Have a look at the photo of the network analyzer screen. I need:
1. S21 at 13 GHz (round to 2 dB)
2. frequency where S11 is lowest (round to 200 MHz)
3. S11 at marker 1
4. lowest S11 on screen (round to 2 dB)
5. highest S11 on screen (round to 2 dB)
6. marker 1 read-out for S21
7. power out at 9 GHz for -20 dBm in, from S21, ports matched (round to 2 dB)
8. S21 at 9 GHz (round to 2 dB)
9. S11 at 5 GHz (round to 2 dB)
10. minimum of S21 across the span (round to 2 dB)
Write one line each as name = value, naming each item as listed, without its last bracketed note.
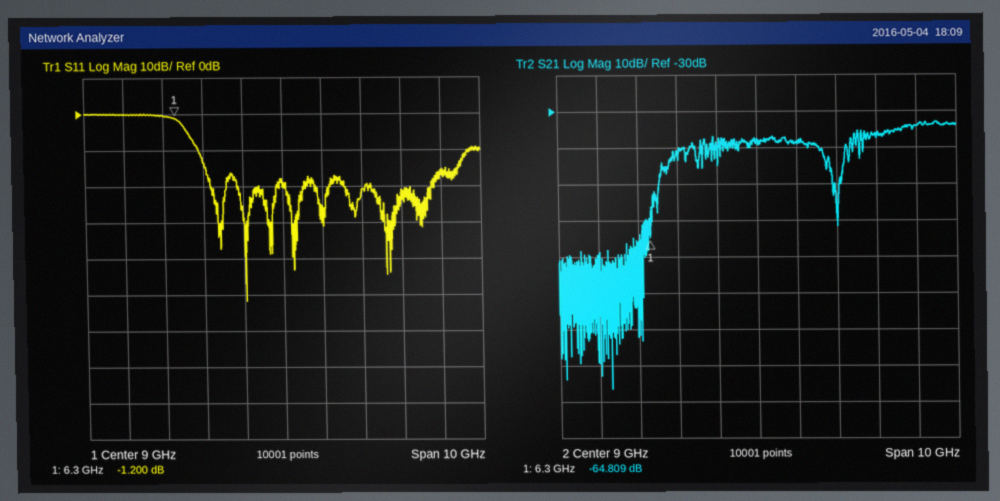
S21 at 13 GHz = -34 dB
frequency where S11 is lowest = 8.0 GHz
S11 at marker 1 = -1.200 dB
lowest S11 on screen = -52 dB
highest S11 on screen = 0 dB
marker 1 read-out for S21 = -64.809 dB
power out at 9 GHz for -20 dBm in, from S21, ports matched = -58 dBm
S21 at 9 GHz = -38 dB
S11 at 5 GHz = 0 dB
minimum of S21 across the span = -106 dB
